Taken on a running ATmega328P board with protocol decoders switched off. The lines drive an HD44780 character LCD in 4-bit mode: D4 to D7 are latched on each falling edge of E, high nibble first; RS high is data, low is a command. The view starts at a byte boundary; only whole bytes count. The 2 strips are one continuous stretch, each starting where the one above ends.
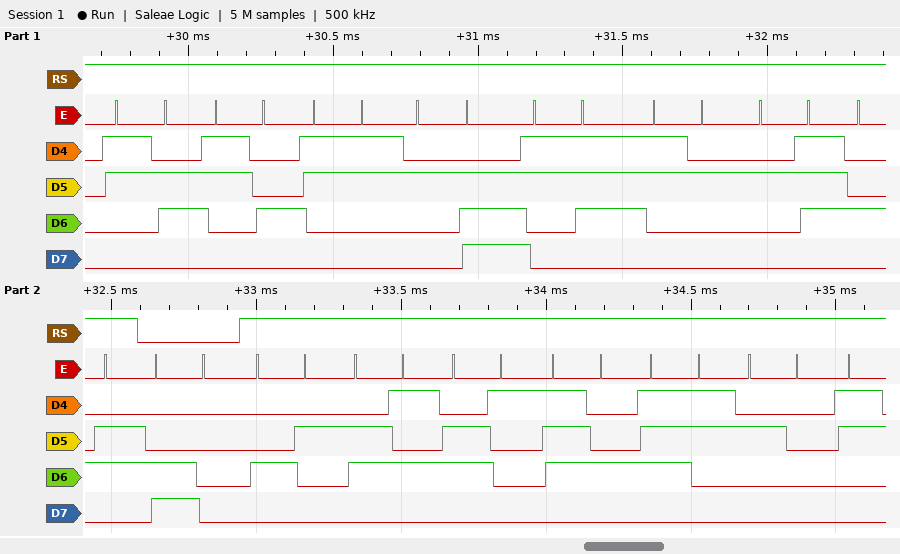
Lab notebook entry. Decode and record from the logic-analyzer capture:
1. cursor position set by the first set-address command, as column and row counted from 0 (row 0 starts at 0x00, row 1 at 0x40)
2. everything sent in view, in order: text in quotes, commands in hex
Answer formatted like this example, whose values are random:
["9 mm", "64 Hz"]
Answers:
["column 0, row 1", "\"643.72'F\" 0xC0 \"Beats \""]
